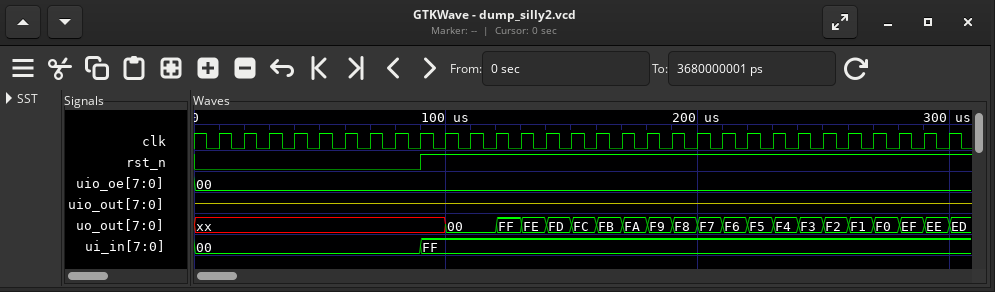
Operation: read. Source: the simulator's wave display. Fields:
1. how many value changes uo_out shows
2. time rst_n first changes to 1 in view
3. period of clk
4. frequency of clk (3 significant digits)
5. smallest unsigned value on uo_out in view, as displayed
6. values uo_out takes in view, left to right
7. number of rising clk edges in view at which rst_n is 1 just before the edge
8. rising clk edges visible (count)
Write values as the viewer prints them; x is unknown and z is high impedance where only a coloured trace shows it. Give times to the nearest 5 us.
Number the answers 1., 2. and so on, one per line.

1. 20
2. 90 us
3. 10 us
4. 100 kHz
5. 00
6. xx, 00, FF, FE, FD, FC, FB, FA, F9, F8, F7, F6, F5, F4, F3, F2, F1, F0, EF, EE, ED
7. 21
8. 30
